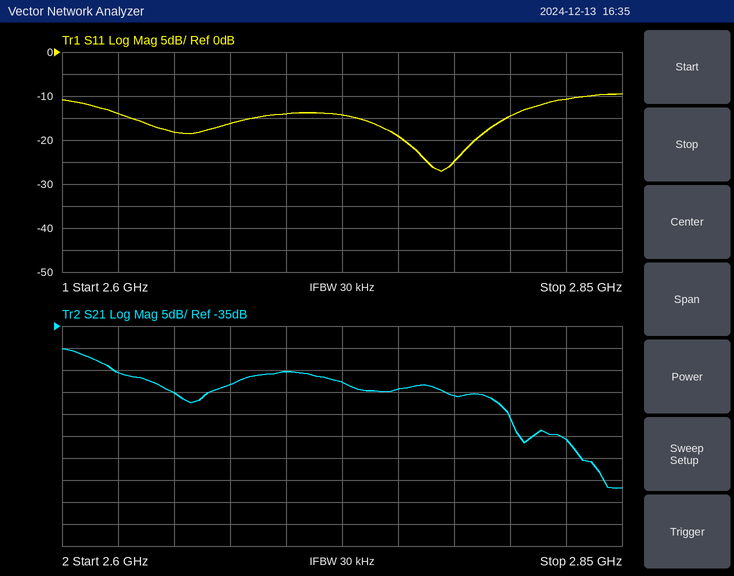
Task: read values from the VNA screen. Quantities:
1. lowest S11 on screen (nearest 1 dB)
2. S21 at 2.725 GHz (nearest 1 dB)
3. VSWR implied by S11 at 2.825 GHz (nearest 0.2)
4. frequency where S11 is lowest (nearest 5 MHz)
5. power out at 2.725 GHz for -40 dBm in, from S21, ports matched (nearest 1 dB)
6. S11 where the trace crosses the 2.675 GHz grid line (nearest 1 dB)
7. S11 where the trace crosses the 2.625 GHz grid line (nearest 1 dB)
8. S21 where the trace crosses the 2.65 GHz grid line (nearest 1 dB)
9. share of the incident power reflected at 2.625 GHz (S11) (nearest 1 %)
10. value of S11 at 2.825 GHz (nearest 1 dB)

-27 dB
-48 dB
1.8
2.770 GHz
-88 dBm
-16 dB
-14 dB
-50 dB
4 %
-11 dB
